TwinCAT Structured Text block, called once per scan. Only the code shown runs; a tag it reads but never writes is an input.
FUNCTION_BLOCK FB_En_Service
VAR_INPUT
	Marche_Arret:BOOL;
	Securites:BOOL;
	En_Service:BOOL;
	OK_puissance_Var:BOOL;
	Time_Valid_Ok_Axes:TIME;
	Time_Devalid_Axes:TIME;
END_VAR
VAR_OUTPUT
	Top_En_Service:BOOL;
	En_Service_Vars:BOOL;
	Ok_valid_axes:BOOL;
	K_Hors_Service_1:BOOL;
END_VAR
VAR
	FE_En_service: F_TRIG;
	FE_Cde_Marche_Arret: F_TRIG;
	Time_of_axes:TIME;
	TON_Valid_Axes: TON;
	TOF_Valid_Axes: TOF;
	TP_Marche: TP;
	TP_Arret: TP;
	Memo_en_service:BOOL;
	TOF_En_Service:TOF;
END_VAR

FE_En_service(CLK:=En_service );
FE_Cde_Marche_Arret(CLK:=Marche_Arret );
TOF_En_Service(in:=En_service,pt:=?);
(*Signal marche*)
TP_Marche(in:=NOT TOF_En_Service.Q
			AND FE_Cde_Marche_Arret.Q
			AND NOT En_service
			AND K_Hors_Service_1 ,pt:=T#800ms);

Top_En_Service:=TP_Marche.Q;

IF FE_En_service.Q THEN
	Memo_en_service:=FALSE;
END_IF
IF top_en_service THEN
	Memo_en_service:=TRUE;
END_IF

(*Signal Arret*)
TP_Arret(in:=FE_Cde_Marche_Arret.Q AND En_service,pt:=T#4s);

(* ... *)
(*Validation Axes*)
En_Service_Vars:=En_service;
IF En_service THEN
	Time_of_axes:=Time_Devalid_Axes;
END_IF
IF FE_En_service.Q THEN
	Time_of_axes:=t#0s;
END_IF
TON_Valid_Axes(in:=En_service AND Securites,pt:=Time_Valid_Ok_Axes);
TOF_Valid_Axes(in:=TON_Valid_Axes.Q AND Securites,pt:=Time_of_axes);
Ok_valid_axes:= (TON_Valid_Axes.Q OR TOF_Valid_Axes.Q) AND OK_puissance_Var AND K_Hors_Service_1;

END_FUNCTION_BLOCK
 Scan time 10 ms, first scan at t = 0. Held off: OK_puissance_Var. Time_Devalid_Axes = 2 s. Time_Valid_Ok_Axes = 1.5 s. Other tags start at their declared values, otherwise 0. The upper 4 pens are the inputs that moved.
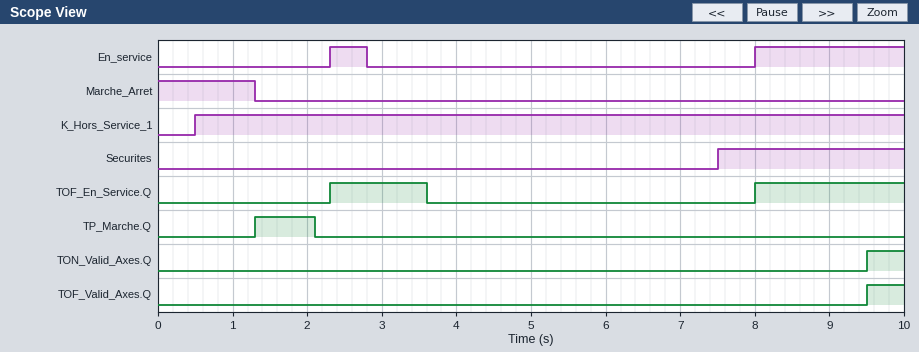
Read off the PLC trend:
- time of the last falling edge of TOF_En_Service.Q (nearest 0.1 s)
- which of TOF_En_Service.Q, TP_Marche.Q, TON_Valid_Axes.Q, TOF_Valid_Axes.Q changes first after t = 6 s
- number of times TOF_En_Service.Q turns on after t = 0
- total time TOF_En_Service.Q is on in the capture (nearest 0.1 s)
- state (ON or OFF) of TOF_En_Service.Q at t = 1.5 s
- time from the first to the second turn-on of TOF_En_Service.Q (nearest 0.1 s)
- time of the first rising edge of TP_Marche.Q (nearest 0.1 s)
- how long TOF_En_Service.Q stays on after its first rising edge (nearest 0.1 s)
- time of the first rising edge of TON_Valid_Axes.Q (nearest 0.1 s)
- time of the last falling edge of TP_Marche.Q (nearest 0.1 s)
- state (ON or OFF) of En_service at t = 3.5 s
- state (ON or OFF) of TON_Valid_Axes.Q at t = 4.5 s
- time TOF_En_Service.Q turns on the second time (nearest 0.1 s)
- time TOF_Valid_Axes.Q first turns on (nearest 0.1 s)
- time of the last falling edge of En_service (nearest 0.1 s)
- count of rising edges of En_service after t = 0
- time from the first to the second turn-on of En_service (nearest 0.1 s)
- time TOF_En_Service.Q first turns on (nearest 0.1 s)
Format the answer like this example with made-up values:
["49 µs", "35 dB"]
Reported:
["3.6 s", "TOF_En_Service.Q", "2", "3.3 s", "OFF", "5.7 s", "1.3 s", "1.3 s", "9.5 s", "2.1 s", "OFF", "OFF", "8.0 s", "9.5 s", "2.8 s", "2", "5.7 s", "2.3 s"]
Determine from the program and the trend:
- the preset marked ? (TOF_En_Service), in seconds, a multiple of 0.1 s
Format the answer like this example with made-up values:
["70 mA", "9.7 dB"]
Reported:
["0.8 s"]
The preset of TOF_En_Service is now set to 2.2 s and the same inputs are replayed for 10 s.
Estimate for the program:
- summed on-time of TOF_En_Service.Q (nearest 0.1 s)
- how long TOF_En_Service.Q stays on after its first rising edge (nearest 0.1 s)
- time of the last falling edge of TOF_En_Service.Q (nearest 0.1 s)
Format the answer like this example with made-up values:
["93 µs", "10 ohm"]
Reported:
["4.7 s", "2.7 s", "5.0 s"]
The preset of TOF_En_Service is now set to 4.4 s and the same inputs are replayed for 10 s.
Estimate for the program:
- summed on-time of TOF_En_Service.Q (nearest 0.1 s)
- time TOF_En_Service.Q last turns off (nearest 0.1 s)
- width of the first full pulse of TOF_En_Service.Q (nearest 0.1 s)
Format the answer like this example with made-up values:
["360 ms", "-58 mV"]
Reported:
["6.9 s", "7.2 s", "4.9 s"]
